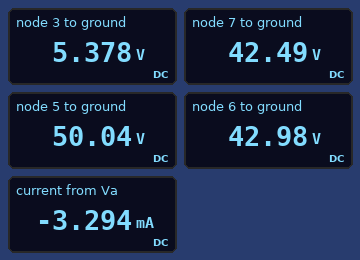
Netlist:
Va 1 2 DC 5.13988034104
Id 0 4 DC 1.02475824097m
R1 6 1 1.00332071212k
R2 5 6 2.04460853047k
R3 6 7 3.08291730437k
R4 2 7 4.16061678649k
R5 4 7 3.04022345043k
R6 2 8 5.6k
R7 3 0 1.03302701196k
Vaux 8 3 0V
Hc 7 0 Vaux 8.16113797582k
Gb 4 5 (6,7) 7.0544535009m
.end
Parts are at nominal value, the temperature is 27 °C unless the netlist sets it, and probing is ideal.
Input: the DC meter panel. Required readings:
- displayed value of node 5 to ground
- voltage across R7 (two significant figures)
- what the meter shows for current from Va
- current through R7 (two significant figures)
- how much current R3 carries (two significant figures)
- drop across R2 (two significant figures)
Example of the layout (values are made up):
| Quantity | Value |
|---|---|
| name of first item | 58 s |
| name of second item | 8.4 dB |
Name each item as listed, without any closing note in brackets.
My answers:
| Quantity | Value |
|---|---|
| displayed value of node 5 to ground | 50.04 V |
| voltage across R7 | 5.4 V |
| what the meter shows for current from Va | -3.294 mA |
| current through R7 | 5.2 mA |
| how much current R3 carries | 160 µA |
| drop across R2 | 7.1 V |
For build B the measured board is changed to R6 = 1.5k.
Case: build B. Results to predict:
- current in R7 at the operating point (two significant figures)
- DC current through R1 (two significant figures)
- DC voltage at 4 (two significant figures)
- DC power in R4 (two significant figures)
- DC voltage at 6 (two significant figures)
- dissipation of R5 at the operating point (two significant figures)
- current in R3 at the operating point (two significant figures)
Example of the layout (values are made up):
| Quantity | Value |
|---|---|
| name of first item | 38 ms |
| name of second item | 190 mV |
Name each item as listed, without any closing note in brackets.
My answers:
| Quantity | Value |
|---|---|
| current in R7 at the operating point | 870 µA |
| DC current through R1 | 310 µA |
| DC voltage at 4 | 11 V |
| DC power in R4 | 5.7 mW |
| DC voltage at 6 | 7.0 V |
| dissipation of R5 at the operating point | 5.5 mW |
| current in R3 at the operating point | 15 µA |
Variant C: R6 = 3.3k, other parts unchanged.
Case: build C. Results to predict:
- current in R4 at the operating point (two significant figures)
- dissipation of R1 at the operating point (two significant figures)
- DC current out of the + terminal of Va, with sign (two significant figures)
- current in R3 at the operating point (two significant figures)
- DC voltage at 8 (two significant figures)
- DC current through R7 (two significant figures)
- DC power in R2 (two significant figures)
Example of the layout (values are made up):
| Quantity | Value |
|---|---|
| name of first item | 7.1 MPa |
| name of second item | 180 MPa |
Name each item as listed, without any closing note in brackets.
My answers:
| Quantity | Value |
|---|---|
| current in R4 at the operating point | 1.3 mA |
| dissipation of R1 at the operating point | 12 µW |
| DC current out of the + terminal of Va, with sign | -110 µA |
| current in R3 at the operating point | 5.3 µA |
| DC voltage at 8 | 1.4 V |
| DC current through R7 | 1.4 mA |
| DC power in R2 | 27 µW |
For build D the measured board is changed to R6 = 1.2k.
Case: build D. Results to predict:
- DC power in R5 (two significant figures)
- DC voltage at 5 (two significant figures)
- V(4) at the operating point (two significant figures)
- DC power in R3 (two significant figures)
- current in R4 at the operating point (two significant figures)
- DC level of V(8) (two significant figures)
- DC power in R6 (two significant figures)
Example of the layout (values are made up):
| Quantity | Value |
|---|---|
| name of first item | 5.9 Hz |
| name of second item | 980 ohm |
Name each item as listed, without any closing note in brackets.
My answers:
| Quantity | Value |
|---|---|
| DC power in R5 | 5.9 mW |
| DC voltage at 5 | 5.9 V |
| V(4) at the operating point | 11 V |
| DC power in R3 | 860 nW |
| current in R4 at the operating point | 1.2 mA |
| DC level of V(8) | 840 mV |
| DC power in R6 | 800 µW |
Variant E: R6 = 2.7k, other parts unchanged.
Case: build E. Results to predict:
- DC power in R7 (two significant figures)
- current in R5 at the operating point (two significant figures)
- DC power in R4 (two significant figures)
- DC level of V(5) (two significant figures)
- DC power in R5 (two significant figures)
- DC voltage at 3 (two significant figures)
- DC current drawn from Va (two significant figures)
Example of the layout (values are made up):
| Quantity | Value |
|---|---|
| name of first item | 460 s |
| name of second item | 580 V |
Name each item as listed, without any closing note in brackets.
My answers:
| Quantity | Value |
|---|---|
| DC power in R7 | 1.4 mW |
| current in R5 at the operating point | 1.1 mA |
| DC power in R4 | 6.2 mW |
| DC level of V(5) | 9.2 V |
| DC power in R5 | 3.7 mW |
| DC voltage at 3 | 1.2 V |
| DC current drawn from Va | 74 µA |
